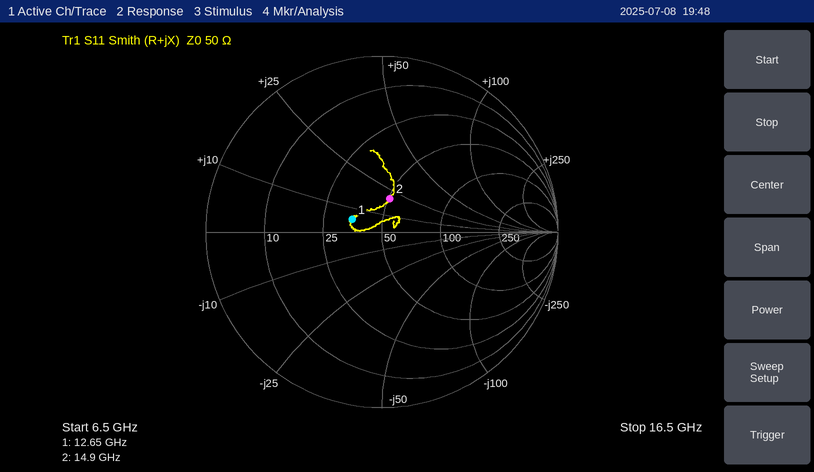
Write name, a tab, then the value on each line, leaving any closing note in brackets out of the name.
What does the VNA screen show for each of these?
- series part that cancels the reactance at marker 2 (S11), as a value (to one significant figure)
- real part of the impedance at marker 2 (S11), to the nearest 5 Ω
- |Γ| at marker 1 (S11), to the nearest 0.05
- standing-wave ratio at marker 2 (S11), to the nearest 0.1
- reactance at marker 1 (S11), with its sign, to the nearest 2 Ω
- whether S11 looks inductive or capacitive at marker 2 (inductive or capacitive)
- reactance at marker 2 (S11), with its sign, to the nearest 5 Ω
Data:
series part that cancels the reactance at marker 2 (S11), as a value	500 fF
real part of the impedance at marker 2 (S11), to the nearest 5 Ω	50 Ω
|Γ| at marker 1 (S11), to the nearest 0.05	0.20
standing-wave ratio at marker 2 (S11), to the nearest 0.1	1.5
reactance at marker 1 (S11), with its sign, to the nearest 2 Ω	+6 Ω
whether S11 looks inductive or capacitive at marker 2	inductive
reactance at marker 2 (S11), with its sign, to the nearest 5 Ω	+20 Ω
